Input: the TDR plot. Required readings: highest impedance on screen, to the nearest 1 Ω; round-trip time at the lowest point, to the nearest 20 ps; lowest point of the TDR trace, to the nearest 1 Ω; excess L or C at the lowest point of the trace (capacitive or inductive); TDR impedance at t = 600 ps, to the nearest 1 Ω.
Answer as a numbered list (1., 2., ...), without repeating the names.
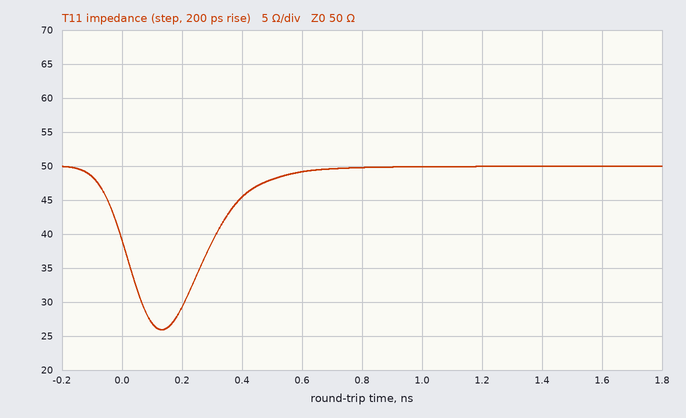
1. 50 Ω
2. 140 ps
3. 26 Ω
4. capacitive
5. 49 Ω
